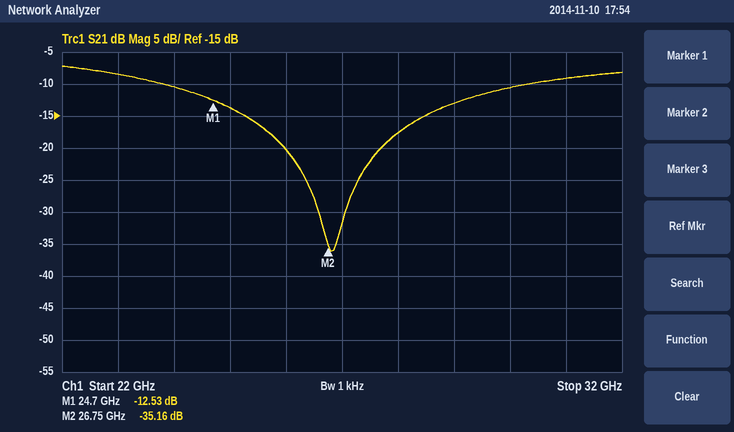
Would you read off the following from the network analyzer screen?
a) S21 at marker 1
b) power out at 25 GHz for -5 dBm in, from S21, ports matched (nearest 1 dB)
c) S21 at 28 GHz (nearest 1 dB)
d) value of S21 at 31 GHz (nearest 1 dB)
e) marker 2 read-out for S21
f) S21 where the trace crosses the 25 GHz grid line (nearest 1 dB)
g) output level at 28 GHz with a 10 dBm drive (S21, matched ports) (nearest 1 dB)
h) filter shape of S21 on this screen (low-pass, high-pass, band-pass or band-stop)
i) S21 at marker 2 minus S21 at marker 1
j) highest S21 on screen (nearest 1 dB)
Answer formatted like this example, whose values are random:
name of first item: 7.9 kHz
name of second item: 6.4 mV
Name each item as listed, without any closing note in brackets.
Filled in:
S21 at marker 1: -12.53 dB
power out at 25 GHz for -5 dBm in, from S21, ports matched: -19 dBm
S21 at 28 GHz: -18 dB
value of S21 at 31 GHz: -9 dB
marker 2 read-out for S21: -35.16 dB
S21 where the trace crosses the 25 GHz grid line: -14 dB
output level at 28 GHz with a 10 dBm drive (S21, matched ports): -8 dBm
filter shape of S21 on this screen: band-stop
S21 at marker 2 minus S21 at marker 1: -22.63 dB
highest S21 on screen: -7 dB
